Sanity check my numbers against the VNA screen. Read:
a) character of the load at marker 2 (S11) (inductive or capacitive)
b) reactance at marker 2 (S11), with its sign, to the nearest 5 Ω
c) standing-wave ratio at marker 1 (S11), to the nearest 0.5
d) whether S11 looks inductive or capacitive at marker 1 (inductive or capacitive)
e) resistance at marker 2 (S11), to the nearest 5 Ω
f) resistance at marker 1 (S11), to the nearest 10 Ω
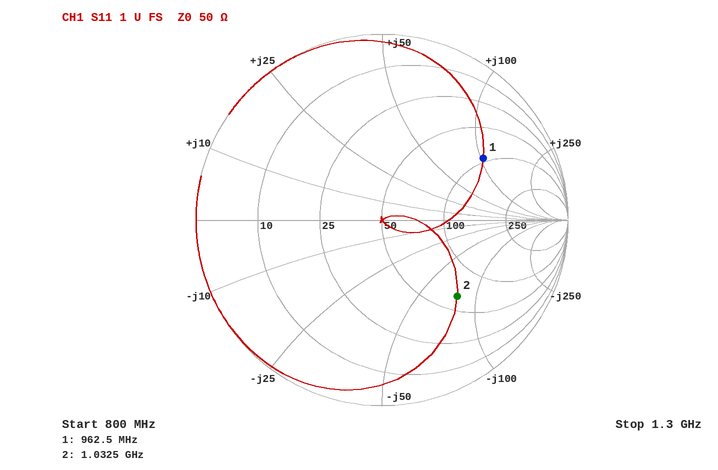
capacitive
-80 Ω
4.5
inductive
65 Ω
90 Ω
